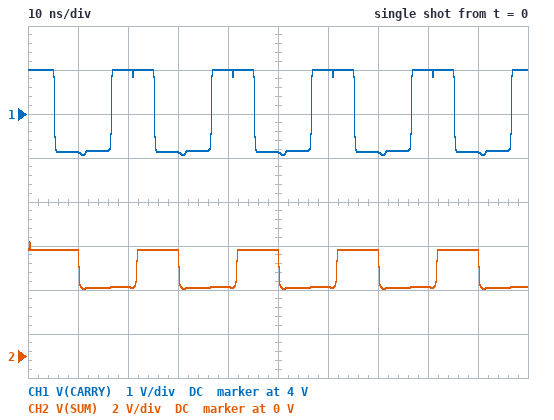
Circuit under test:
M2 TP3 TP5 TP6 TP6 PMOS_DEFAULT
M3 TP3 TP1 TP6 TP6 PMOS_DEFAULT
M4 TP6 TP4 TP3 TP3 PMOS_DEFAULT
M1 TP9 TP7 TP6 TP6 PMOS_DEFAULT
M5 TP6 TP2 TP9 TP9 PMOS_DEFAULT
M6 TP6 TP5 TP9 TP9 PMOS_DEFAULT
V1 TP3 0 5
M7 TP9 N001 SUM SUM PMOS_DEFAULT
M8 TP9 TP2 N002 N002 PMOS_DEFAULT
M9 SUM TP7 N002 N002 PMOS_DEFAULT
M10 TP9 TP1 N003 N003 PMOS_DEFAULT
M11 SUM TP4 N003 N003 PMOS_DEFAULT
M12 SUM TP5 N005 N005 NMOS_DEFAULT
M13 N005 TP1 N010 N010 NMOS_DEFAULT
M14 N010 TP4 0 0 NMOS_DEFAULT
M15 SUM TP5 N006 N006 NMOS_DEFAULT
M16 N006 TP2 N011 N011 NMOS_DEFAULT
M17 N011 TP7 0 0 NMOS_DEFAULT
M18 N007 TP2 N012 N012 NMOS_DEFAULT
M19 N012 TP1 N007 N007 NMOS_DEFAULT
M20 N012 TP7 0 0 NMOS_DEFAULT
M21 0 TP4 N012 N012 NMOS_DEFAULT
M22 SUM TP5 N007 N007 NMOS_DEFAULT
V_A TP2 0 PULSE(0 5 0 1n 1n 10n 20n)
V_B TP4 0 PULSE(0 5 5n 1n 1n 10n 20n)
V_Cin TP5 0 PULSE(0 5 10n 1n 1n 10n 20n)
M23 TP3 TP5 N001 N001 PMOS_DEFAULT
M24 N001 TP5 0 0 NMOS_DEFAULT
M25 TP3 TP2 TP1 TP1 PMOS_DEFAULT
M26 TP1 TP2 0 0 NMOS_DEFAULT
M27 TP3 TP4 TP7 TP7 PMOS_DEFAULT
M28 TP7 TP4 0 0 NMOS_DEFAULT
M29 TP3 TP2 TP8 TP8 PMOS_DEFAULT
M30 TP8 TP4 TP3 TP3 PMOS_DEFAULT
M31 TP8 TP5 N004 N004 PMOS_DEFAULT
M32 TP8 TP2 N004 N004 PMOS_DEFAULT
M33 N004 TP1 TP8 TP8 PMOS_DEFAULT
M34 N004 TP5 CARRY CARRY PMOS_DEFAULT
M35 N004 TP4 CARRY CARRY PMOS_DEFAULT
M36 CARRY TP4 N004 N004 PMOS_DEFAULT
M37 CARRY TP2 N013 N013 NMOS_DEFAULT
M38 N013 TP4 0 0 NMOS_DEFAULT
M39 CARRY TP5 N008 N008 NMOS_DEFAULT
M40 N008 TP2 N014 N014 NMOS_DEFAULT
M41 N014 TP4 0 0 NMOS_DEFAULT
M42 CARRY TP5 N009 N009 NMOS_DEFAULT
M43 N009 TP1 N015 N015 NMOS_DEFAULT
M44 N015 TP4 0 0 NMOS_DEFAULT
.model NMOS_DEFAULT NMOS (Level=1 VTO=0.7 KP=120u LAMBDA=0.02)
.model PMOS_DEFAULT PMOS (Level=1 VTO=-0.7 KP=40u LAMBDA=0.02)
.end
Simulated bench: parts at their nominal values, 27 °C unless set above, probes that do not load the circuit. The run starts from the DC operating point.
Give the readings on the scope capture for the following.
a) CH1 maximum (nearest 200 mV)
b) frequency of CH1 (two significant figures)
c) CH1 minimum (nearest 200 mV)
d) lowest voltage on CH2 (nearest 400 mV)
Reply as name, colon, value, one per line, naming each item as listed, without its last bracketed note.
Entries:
CH1 maximum: 5.0 V
frequency of CH1: 50 MHz
CH1 minimum: 3.0 V
lowest voltage on CH2: 3.2 V
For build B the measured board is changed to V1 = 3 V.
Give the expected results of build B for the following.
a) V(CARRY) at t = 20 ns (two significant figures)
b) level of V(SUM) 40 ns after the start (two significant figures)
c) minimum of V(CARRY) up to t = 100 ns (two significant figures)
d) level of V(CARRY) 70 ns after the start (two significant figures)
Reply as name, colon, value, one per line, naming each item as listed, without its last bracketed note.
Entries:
V(CARRY) at t = 20 ns: 3.0 V
level of V(SUM) 40 ns after the start: 1.3 V
minimum of V(CARRY) up to t = 100 ns: 1.1 V
level of V(CARRY) 70 ns after the start: 1.2 V
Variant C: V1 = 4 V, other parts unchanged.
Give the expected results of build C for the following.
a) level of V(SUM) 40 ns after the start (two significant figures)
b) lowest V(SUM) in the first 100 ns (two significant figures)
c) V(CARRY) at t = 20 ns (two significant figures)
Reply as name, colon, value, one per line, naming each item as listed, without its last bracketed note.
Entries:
level of V(SUM) 40 ns after the start: 2.2 V
lowest V(SUM) in the first 100 ns: 2.1 V
V(CARRY) at t = 20 ns: 4.0 V
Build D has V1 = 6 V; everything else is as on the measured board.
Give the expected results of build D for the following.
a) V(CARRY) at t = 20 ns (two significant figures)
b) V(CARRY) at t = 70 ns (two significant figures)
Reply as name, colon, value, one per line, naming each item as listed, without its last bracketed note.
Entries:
V(CARRY) at t = 20 ns: 6.0 V
V(CARRY) at t = 70 ns: 4.1 V
